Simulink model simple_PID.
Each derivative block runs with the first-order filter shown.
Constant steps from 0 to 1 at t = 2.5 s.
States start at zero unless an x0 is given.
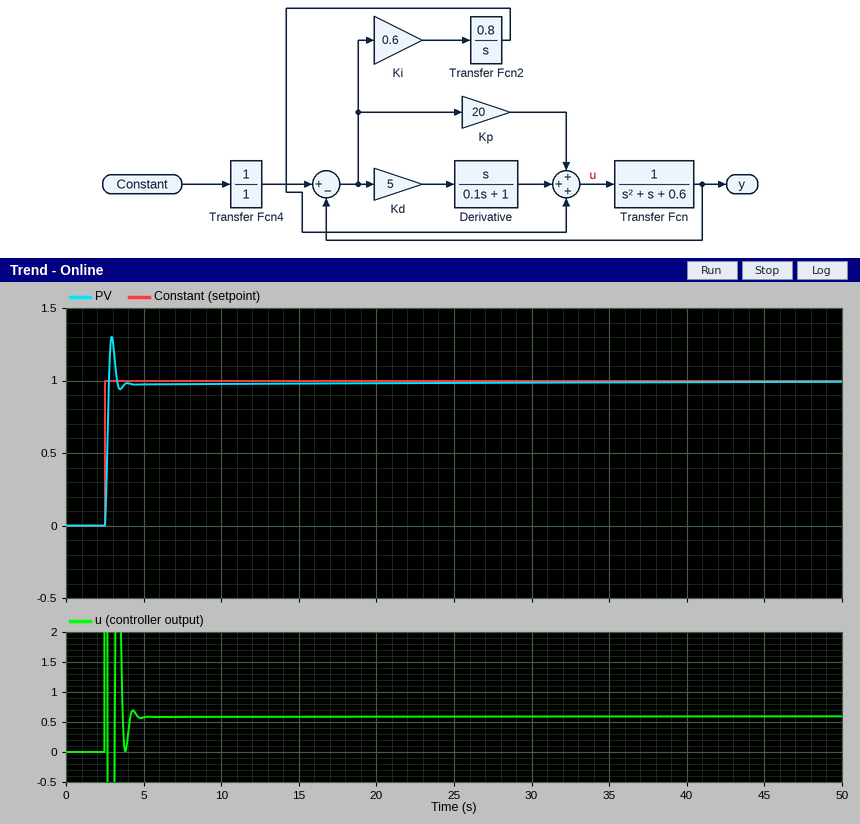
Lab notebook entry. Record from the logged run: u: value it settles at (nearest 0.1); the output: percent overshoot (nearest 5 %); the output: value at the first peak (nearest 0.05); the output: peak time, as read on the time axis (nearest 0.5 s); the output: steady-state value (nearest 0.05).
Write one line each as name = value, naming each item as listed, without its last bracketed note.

u: value it settles at = 0.6
the output: percent overshoot = 30 %
the output: value at the first peak = 1.30
the output: peak time, as read on the time axis = 3.0 s
the output: steady-state value = 1.00
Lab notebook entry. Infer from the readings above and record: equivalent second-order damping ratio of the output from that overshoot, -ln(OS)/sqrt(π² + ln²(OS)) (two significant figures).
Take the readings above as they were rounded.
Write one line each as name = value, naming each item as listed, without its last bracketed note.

equivalent second-order damping ratio of the output from that overshoot, -ln(OS)/sqrt(π² + ln²(OS)) = 0.36
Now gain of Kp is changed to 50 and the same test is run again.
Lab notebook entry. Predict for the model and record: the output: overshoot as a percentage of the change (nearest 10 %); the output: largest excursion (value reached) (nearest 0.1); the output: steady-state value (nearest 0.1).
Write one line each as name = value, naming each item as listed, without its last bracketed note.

the output: overshoot as a percentage of the change = 50 %
the output: largest excursion (value reached) = 1.5
the output: steady-state value = 1.0
